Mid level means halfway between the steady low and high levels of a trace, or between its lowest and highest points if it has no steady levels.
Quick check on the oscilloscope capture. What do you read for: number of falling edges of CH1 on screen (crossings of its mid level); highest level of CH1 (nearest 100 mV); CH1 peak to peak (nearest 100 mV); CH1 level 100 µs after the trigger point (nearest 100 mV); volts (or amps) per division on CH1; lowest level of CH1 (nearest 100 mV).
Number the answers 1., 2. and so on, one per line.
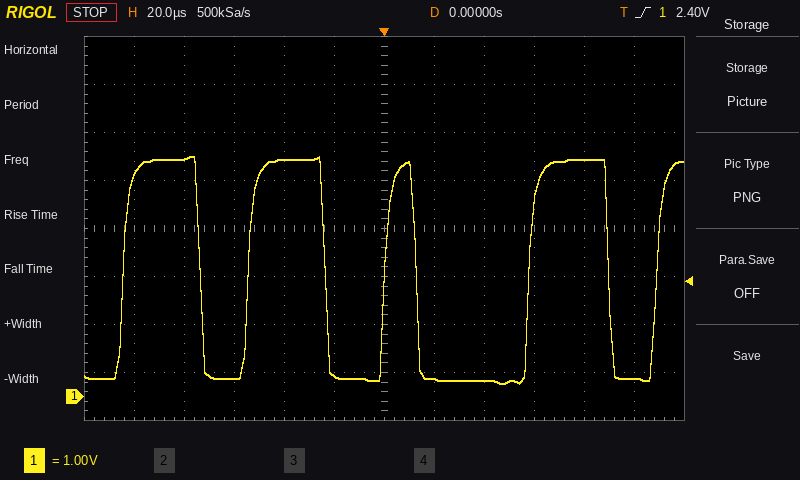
1. 4
2. 5.0 V
3. 4.7 V
4. 400 mV
5. 1 V
6. 300 mV
